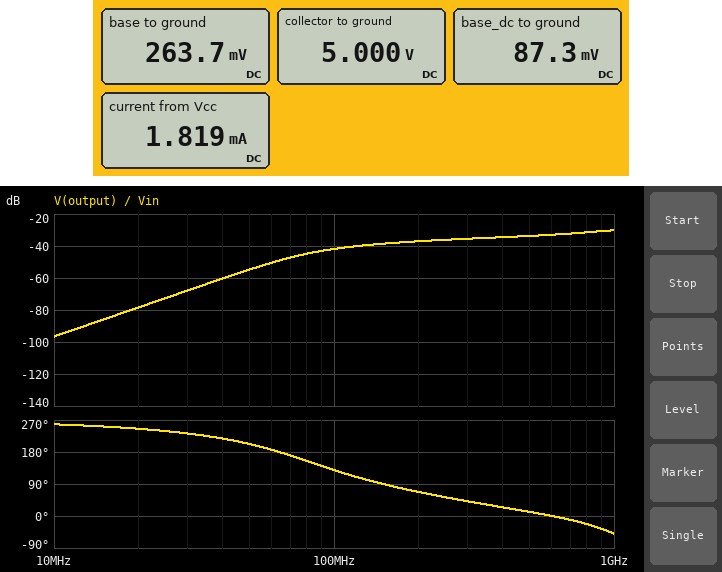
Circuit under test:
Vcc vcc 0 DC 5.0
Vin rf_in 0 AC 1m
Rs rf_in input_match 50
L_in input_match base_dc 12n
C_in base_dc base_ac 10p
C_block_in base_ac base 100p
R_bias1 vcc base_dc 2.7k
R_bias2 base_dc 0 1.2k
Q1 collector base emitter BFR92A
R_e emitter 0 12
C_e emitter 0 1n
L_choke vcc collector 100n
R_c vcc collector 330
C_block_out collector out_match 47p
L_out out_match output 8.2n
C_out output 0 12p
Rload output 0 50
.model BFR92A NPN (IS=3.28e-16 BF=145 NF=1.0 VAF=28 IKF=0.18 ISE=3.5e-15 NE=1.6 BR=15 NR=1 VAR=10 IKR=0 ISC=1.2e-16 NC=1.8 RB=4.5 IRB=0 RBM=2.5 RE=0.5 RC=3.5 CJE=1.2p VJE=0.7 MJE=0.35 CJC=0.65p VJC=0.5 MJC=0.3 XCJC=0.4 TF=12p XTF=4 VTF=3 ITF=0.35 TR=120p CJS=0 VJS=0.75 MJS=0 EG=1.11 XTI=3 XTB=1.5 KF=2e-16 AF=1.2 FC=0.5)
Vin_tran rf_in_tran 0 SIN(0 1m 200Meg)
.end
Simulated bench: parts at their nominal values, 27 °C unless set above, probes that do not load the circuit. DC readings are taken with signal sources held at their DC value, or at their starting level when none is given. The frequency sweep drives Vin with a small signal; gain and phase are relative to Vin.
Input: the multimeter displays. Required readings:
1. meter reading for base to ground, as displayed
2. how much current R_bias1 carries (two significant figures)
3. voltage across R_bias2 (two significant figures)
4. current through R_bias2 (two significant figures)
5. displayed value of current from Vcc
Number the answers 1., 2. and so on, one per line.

1. 263.7 mV
2. 1.8 mA
3. 87 mV
4. 73 µA
5. 1.819 mA
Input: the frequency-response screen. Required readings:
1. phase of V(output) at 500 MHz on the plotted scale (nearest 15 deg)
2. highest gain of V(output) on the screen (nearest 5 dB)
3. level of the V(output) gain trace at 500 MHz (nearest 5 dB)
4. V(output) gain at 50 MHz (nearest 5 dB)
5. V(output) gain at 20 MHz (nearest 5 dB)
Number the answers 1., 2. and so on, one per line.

1. 15 deg
2. -30 dB
3. -35 dB
4. -55 dB
5. -80 dB
